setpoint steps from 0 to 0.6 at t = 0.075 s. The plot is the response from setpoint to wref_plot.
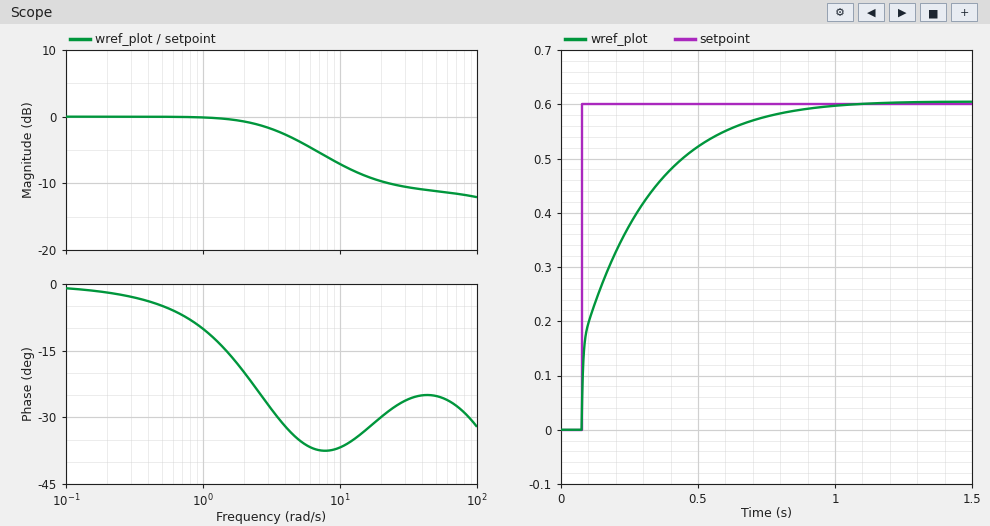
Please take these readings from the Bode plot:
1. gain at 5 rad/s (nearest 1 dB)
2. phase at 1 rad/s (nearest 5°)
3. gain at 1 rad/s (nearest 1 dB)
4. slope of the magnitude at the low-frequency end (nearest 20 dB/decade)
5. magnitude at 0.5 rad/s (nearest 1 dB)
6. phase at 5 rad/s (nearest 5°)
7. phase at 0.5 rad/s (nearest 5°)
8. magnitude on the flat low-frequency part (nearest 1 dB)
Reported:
-4 dB
-10°
0 dB
0 dB/decade
0 dB
-35°
-5°
0 dB
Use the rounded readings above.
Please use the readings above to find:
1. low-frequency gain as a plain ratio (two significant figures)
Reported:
1.0
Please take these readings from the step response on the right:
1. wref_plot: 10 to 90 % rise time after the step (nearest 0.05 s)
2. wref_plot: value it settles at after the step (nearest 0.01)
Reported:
0.50 s
0.60
